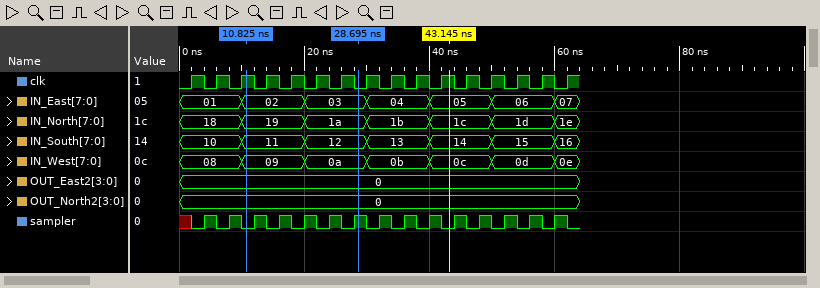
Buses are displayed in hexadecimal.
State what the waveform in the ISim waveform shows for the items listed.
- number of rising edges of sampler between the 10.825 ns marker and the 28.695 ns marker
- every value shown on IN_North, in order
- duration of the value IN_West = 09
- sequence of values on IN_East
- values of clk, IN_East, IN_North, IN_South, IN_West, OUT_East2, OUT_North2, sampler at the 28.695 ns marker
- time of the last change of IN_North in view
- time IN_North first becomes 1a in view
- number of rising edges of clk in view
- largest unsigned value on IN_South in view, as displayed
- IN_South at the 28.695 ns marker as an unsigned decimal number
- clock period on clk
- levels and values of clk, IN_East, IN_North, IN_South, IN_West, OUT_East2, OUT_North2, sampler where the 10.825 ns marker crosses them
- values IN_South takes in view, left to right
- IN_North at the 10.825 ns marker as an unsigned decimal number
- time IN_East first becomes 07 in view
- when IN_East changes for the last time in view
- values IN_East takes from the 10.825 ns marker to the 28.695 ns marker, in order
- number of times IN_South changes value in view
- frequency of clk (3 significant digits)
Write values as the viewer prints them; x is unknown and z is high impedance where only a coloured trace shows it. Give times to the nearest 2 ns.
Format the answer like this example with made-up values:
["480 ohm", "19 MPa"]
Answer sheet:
["5", "18, 19, 1a, 1b, 1c, 1d, 1e", "10 ns", "01, 02, 03, 04, 05, 06, 07", "clk=0, IN_East=03, IN_North=1a, IN_South=12, IN_West=0a, OUT_East2=0, OUT_North2=0, sampler=1", "60 ns", "20 ns", "16", "16", "18", "4 ns", "clk=1, IN_East=02, IN_North=19, IN_South=11, IN_West=09, OUT_East2=0, OUT_North2=0, sampler=0", "10, 11, 12, 13, 14, 15, 16", "25", "60 ns", "60 ns", "02, 03", "6", "250 MHz"]
